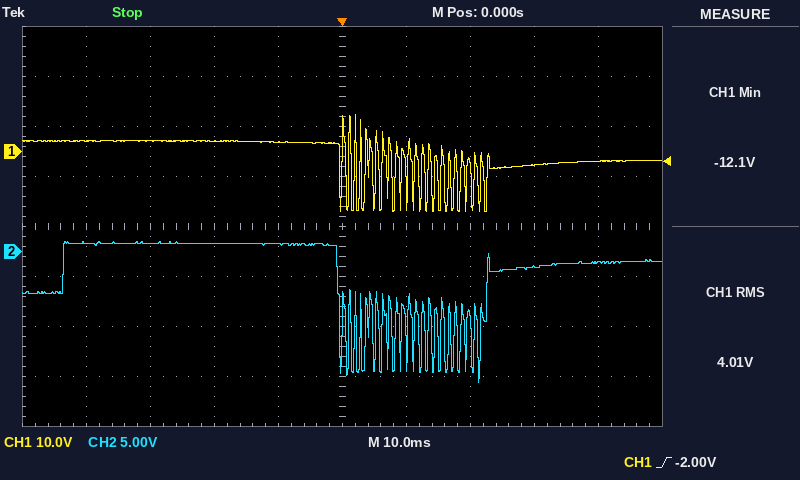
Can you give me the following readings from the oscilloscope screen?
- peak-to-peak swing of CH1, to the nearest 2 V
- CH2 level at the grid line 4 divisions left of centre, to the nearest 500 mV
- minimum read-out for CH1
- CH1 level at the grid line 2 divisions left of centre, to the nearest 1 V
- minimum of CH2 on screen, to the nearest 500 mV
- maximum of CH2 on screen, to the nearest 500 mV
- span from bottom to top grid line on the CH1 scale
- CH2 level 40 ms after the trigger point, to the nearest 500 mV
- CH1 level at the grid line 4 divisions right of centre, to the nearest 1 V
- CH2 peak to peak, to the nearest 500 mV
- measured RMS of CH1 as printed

20 V
1.0 V
-12.1 V
2 V
-13.0 V
1.0 V
80 V
-1.0 V
-2 V
14.0 V
4.01 V
